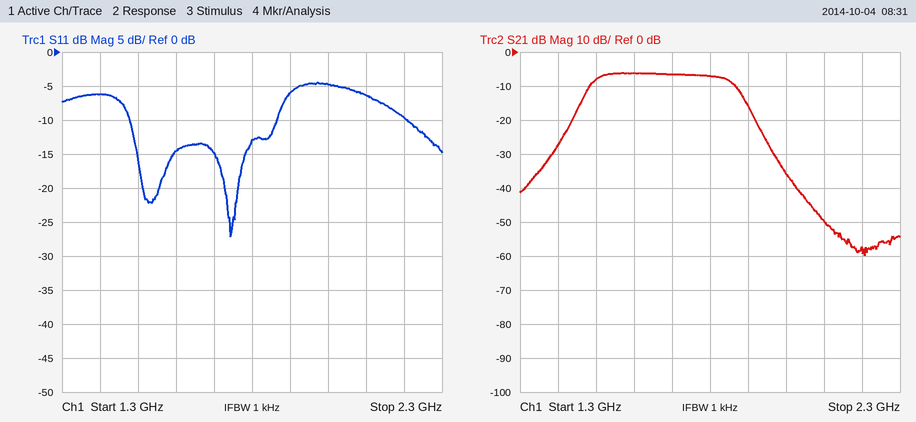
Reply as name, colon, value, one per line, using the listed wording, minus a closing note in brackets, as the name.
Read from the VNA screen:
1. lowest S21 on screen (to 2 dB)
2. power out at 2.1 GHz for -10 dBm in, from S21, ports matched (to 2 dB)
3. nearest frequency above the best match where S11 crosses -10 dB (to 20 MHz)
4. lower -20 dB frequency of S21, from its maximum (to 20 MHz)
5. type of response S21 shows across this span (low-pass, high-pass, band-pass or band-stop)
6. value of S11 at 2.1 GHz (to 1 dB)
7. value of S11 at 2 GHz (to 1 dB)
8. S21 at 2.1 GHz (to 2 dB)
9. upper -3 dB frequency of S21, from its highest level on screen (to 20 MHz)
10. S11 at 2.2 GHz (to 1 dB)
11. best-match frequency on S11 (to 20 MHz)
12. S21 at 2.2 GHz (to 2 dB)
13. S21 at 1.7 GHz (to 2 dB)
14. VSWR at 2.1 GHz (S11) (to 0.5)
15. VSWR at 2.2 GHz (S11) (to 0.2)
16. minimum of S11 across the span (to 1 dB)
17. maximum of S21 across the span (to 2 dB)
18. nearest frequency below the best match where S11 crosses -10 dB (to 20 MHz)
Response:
lowest S21 on screen: -60 dB
power out at 2.1 GHz for -10 dBm in, from S21, ports matched: -60 dBm
nearest frequency above the best match where S11 crosses -10 dB: 1.86 GHz
lower -20 dB frequency of S21, from its maximum: 1.40 GHz
type of response S21 shows across this span: band-pass
value of S11 at 2.1 GHz: -6 dB
value of S11 at 2 GHz: -5 dB
S21 at 2.1 GHz: -50 dB
upper -3 dB frequency of S21, from its highest level on screen: 1.86 GHz
S11 at 2.2 GHz: -10 dB
best-match frequency on S11: 1.74 GHz
S21 at 2.2 GHz: -58 dB
S21 at 1.7 GHz: -6 dB
VSWR at 2.1 GHz (S11): 3.0
VSWR at 2.2 GHz (S11): 2.0
minimum of S11 across the span: -27 dB
maximum of S21 across the span: -6 dB
nearest frequency below the best match where S11 crosses -10 dB: 1.48 GHz
